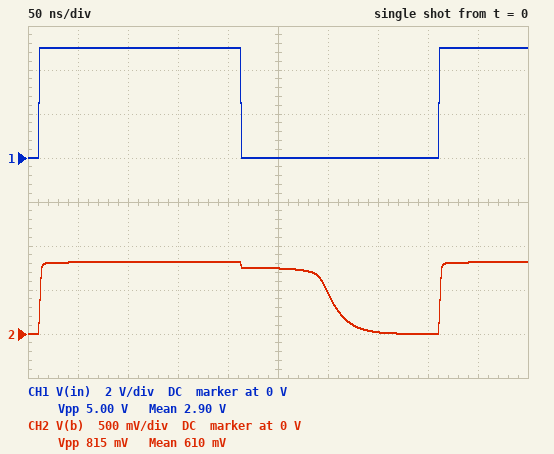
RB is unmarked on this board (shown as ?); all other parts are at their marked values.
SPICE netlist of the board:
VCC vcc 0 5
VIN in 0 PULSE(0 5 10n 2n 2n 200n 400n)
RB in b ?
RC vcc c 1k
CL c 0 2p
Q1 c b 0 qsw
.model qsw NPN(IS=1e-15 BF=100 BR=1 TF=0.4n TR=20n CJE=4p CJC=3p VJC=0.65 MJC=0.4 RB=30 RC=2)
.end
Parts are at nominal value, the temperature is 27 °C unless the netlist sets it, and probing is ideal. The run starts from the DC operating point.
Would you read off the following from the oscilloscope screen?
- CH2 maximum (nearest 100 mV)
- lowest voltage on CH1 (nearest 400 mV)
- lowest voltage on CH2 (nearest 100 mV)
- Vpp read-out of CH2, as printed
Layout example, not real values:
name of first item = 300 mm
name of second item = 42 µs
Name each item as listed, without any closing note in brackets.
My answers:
CH2 maximum = 800 mV
lowest voltage on CH1 = 0 V
lowest voltage on CH2 = 0 V
Vpp read-out of CH2, as printed = 815 mV
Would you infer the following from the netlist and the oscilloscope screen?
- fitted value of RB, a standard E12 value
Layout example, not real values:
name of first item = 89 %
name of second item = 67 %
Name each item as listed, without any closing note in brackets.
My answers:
fitted value of RB, a standard E12 value = 2.7 kΩ
